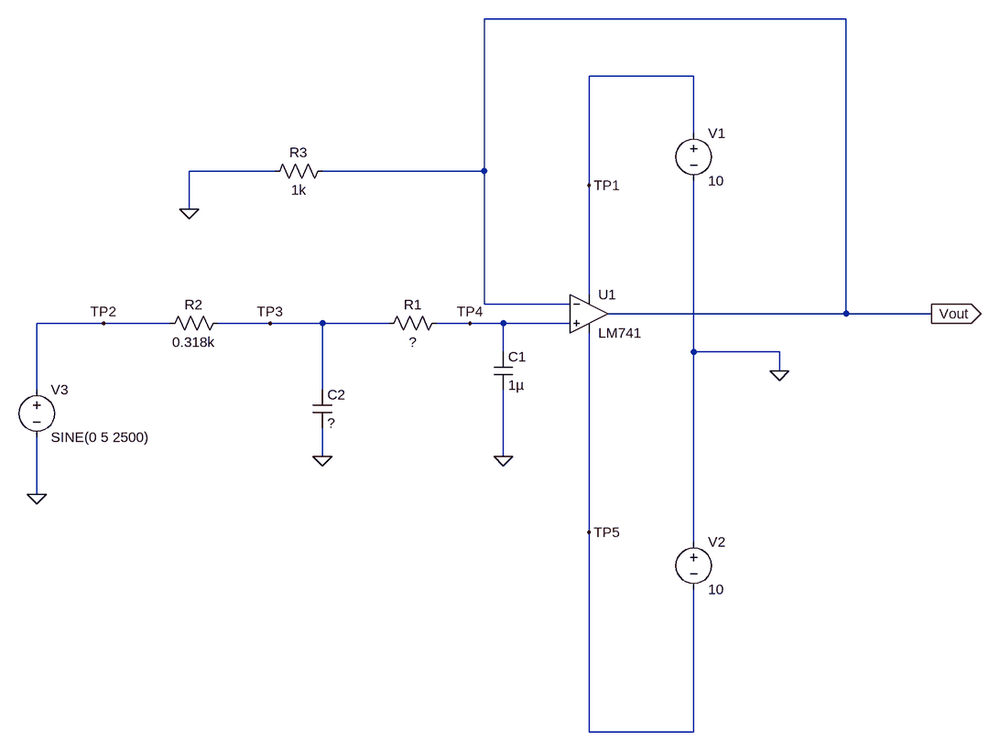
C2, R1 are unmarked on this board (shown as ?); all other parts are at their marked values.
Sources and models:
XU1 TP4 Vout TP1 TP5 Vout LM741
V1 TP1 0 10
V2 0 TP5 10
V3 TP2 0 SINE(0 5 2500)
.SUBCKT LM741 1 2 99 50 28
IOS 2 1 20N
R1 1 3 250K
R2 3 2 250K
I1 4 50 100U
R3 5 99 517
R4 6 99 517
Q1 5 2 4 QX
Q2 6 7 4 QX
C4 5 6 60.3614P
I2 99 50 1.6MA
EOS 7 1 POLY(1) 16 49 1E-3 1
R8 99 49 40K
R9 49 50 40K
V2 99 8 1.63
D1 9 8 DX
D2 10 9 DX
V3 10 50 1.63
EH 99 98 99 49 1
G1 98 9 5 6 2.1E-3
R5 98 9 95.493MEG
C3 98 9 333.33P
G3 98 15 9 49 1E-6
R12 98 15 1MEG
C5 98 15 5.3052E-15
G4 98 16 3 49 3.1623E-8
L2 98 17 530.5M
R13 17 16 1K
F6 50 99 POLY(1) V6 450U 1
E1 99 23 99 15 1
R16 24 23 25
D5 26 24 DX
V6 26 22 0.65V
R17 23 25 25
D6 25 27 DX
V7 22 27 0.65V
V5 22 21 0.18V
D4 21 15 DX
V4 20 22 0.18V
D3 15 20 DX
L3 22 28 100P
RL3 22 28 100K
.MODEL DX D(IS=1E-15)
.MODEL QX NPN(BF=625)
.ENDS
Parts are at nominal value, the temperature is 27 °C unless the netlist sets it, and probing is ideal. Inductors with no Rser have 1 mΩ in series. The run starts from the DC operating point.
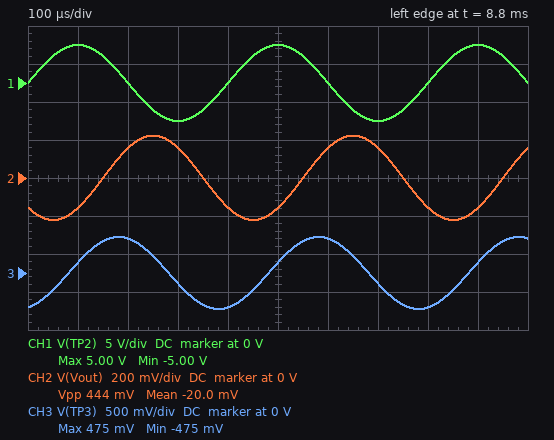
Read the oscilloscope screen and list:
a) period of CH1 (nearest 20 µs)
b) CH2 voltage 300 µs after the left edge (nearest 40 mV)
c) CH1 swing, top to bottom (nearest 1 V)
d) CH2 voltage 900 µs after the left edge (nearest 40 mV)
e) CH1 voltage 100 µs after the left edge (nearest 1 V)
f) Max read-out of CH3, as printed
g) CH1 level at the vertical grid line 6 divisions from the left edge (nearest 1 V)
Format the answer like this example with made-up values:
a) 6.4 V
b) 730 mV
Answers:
a) 400 µs
b) 160 mV
c) 10 V
d) -160 mV
e) 5 V
f) 475 mV
g) 0 V
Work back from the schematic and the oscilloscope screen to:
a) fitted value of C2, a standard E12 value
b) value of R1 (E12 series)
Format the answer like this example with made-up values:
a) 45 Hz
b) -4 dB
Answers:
a) 1.8 µF
b) 120 Ω
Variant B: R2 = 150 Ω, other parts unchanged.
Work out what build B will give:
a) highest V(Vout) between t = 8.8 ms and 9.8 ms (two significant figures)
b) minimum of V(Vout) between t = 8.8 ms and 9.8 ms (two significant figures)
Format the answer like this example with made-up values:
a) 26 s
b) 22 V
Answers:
a) 460 mV
b) -450 mV
